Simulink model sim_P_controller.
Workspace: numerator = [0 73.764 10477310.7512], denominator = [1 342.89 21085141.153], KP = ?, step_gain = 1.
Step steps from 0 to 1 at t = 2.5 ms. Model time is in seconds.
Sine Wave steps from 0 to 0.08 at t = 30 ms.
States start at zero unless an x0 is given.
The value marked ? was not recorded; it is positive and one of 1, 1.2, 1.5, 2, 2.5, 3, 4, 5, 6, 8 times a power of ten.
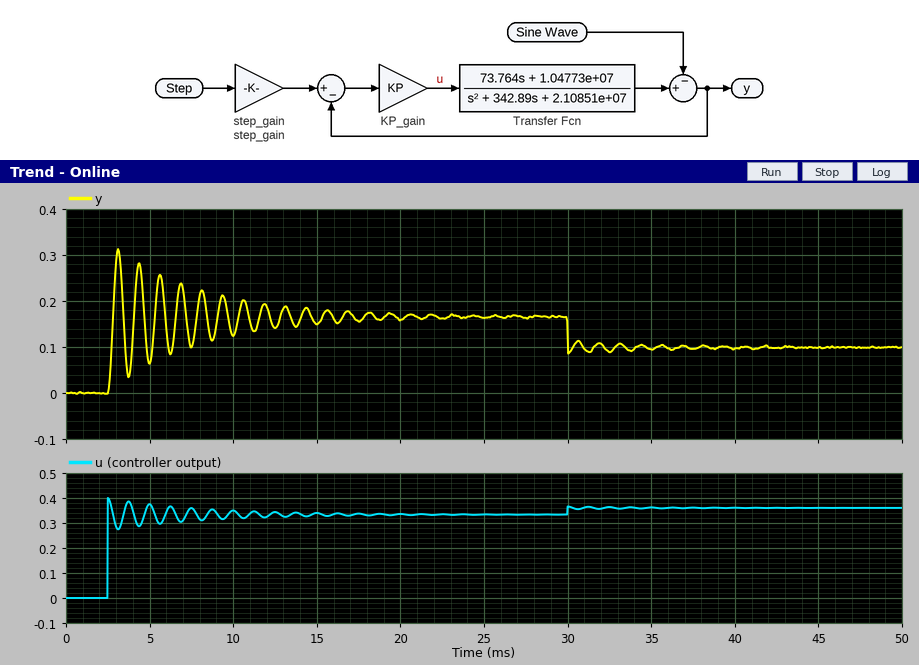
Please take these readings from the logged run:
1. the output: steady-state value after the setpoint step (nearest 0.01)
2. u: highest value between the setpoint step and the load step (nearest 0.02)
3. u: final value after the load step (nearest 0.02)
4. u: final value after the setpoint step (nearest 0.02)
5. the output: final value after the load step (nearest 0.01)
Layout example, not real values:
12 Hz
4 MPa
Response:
0.17
0.40
0.36
0.34
0.10
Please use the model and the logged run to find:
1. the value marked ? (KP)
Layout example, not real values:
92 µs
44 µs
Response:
0.4
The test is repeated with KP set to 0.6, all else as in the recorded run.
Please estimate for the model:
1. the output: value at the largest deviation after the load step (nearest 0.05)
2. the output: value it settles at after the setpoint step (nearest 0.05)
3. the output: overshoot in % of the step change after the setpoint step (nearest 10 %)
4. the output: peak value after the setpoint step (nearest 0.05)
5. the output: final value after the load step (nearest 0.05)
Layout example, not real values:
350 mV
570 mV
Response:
0.15
0.25
90 %
0.45
0.15
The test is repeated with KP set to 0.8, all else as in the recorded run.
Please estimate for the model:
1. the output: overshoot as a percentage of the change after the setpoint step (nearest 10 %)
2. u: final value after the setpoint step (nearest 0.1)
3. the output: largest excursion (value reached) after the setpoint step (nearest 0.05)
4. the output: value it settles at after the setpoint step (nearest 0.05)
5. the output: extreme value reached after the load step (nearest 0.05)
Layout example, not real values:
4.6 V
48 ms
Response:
90 %
0.6
0.55
0.30
0.20
